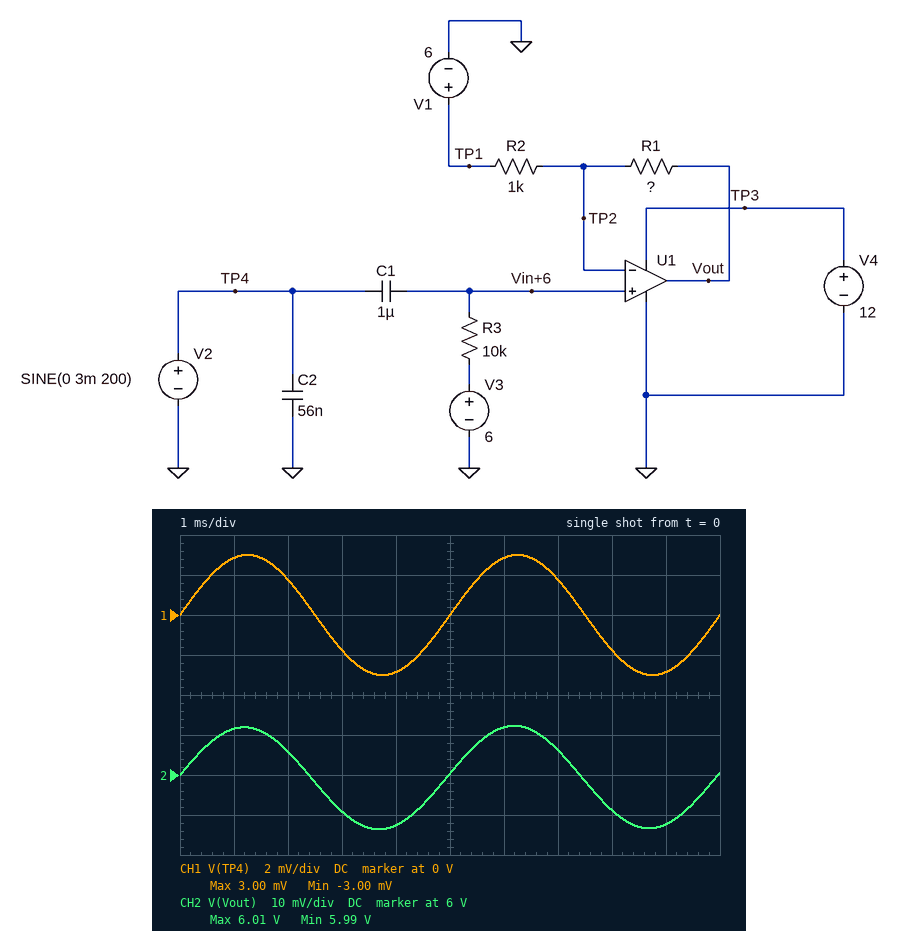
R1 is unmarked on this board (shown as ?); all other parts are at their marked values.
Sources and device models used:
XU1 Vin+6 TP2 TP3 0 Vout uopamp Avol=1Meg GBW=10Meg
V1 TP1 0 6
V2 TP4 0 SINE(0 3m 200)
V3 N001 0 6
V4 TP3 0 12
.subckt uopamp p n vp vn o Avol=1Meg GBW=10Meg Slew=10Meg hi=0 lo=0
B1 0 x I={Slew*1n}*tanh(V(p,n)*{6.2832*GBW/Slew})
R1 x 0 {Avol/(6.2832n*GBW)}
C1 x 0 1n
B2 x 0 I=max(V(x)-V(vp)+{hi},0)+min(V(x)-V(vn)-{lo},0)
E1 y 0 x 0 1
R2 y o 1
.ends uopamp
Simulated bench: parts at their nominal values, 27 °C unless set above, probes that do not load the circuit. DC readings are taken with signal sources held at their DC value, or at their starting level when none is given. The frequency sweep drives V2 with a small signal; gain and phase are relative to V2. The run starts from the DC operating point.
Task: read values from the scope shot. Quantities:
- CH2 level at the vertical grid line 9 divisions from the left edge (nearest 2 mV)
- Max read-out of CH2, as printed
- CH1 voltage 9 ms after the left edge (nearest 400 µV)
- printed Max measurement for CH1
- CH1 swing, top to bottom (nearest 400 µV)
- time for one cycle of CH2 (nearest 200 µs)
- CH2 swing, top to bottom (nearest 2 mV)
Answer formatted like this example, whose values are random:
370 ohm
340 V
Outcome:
5.988 V
6.01 V
-2.8 mV
3.00 mV
6.0 mV
5.0 ms
26 mV
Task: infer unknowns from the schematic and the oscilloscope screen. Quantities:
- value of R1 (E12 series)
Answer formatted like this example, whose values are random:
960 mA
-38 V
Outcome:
3.3 kΩ
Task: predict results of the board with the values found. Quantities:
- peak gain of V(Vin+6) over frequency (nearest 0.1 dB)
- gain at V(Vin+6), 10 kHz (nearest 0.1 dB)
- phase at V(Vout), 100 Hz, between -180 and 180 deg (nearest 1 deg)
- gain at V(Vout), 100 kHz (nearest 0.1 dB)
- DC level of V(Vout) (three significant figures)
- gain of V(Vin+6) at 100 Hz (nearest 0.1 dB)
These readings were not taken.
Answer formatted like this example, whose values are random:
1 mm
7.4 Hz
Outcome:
0 dB
0 dB
9 deg
12.7 dB
6.00 V
-0.1 dB
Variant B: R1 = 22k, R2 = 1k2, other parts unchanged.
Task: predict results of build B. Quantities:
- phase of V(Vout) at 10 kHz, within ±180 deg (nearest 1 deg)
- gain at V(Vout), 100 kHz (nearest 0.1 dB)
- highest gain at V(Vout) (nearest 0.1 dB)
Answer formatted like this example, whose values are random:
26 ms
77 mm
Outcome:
-1 deg
25.6 dB
25.7 dB
